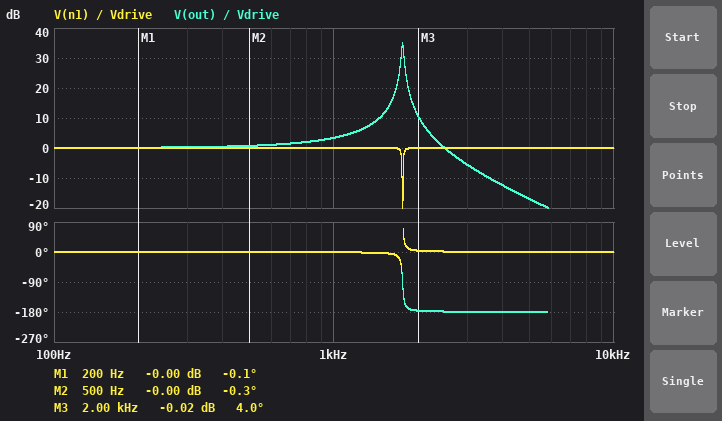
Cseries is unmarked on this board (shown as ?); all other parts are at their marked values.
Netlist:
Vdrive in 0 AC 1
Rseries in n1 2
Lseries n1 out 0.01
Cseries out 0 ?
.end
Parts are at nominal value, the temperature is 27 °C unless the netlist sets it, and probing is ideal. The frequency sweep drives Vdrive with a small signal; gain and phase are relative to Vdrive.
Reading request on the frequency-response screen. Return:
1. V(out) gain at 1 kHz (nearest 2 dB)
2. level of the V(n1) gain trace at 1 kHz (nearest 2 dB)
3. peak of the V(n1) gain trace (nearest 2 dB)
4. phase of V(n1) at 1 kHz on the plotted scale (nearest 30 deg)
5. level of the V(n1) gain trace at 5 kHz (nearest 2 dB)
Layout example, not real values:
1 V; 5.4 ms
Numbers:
4 dB; 0 dB; 0 dB; 0 deg; 0 dB
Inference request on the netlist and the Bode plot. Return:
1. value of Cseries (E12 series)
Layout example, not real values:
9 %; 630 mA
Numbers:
820 nF
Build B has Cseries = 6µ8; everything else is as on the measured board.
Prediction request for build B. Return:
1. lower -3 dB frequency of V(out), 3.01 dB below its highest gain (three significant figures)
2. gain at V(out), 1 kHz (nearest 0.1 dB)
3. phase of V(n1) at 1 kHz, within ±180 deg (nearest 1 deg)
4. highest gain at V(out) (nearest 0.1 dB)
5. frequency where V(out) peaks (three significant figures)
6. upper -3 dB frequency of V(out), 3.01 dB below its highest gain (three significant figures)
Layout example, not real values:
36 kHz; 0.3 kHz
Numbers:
594 Hz; -4.5 dB; 3 deg; 25.7 dB; 610 Hz; 626 Hz
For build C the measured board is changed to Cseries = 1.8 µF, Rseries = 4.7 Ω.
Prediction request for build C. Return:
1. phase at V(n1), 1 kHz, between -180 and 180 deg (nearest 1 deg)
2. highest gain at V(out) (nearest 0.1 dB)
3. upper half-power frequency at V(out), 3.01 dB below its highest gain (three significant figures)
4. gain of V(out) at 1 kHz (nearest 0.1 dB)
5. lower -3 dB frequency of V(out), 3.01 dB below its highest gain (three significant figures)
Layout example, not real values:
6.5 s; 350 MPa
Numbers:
-10 deg; 24.0 dB; 1.22 kHz; 10.6 dB; 1.15 kHz
